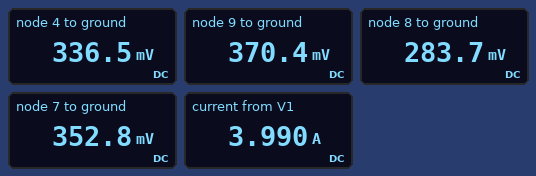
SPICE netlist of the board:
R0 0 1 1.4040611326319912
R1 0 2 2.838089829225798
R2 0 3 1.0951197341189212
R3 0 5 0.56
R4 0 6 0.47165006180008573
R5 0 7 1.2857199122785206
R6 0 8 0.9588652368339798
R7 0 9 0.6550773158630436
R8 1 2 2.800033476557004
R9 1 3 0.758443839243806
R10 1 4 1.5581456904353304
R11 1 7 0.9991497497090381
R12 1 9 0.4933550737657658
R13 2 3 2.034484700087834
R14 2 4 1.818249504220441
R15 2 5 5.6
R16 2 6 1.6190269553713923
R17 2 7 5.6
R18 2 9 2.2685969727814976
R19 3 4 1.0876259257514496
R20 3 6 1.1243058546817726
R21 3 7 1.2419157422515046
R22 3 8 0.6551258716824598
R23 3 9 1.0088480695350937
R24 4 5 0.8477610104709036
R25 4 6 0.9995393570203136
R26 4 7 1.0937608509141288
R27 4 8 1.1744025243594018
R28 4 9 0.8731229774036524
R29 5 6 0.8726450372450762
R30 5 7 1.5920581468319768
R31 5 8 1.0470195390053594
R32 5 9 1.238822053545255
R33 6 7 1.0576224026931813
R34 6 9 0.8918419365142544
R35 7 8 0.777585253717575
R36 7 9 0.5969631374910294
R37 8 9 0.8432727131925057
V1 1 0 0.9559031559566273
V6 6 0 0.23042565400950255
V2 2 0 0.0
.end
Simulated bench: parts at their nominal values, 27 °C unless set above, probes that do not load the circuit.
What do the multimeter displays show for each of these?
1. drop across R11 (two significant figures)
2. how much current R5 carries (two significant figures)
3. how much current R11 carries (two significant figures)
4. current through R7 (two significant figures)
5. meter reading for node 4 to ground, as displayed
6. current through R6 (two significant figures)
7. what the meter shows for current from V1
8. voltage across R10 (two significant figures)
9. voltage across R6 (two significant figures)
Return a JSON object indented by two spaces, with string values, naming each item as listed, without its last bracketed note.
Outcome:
{
  "drop across R11": "600 mV",
  "how much current R5 carries": "270 mA",
  "how much current R11 carries": "600 mA",
  "current through R7": "570 mA",
  "meter reading for node 4 to ground, as displayed": "336.5 mV",
  "current through R6": "300 mA",
  "what the meter shows for current from V1": "3.990 A",
  "voltage across R10": "620 mV",
  "voltage across R6": "280 mV"
}
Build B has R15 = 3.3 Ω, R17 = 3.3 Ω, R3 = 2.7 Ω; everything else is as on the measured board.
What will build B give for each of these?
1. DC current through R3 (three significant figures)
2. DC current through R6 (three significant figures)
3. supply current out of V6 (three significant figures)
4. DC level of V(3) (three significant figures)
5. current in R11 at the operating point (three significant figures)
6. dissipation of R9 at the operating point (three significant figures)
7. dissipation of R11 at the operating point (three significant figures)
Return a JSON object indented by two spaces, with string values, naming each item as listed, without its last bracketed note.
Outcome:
{
  "DC current through R3": "103 mA",
  "DC current through R6": "310 mA",
  "supply current out of V6": "45.4 mA",
  "DC level of V(3)": "370 mV",
  "current in R11 at the operating point": "598 mA",
  "dissipation of R9 at the operating point": "453 mW",
  "dissipation of R11 at the operating point": "358 mW"
}
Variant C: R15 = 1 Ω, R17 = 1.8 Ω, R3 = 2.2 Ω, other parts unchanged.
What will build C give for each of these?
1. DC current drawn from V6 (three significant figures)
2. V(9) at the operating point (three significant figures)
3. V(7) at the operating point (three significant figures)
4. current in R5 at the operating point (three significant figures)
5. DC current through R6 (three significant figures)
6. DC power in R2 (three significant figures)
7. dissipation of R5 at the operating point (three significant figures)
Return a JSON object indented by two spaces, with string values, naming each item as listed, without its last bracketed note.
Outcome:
{
  "DC current drawn from V6": "147 mA",
  "V(9) at the operating point": "369 mV",
  "V(7) at the operating point": "338 mV",
  "current in R5 at the operating point": "263 mA",
  "DC current through R6": "295 mA",
  "DC power in R2": "120 mW",
  "dissipation of R5 at the operating point": "88.8 mW"
}
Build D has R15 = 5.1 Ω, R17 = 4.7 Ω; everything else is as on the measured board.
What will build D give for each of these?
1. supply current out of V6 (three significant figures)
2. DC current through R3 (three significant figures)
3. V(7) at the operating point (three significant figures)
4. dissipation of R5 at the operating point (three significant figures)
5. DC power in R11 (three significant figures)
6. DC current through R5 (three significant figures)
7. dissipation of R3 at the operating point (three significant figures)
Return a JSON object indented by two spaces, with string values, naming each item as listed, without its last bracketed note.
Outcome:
{
  "supply current out of V6": "153 mA",
  "DC current through R3": "386 mA",
  "V(7) at the operating point": "351 mV",
  "dissipation of R5 at the operating point": "95.8 mW",
  "DC power in R11": "366 mW",
  "DC current through R5": "273 mA",
  "dissipation of R3 at the operating point": "83.6 mW"
}
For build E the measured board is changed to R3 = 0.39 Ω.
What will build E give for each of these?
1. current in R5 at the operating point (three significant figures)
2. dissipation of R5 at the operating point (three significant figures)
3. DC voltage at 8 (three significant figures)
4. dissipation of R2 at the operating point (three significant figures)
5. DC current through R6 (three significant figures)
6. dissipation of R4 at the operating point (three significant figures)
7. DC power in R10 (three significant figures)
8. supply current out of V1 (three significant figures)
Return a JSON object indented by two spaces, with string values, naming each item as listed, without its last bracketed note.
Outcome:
{
  "current in R5 at the operating point": "271 mA",
  "dissipation of R5 at the operating point": "94.1 mW",
  "DC voltage at 8": "277 mV",
  "dissipation of R2 at the operating point": "119 mW",
  "DC current through R6": "289 mA",
  "dissipation of R4 at the operating point": "113 mW",
  "DC power in R10": "252 mW",
  "supply current out of V1": "4.01 A"
}
